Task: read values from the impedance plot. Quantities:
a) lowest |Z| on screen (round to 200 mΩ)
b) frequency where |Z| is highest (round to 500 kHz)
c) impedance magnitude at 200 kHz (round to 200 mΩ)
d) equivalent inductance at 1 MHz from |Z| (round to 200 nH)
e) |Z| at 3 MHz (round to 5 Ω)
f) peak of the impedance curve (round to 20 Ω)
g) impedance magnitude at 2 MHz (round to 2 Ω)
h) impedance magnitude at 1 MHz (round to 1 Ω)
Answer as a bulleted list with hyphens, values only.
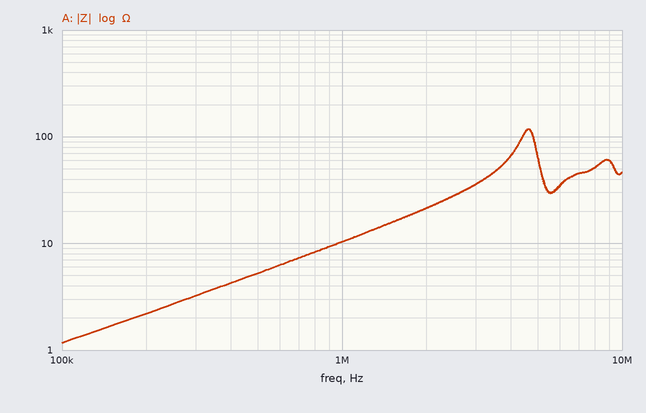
- 1.2 Ω
- 4.5 MHz
- 2.2 Ω
- 1.6 µH
- 35 Ω
- 120 Ω
- 22 Ω
- 10 Ω
